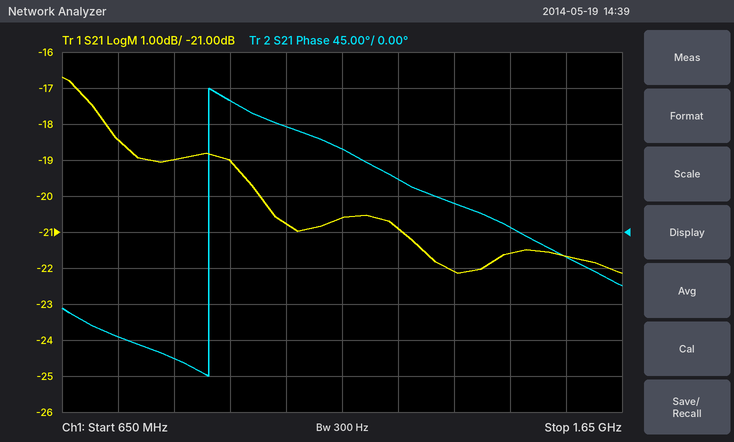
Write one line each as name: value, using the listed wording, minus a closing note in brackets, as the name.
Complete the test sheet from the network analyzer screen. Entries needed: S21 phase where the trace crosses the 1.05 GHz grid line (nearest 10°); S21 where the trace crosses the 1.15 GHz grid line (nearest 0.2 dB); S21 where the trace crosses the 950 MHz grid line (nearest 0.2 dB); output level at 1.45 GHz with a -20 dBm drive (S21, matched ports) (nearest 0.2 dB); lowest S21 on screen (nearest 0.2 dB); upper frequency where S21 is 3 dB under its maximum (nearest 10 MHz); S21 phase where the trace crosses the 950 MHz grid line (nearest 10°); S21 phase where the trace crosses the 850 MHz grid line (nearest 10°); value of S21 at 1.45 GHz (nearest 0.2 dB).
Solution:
S21 phase where the trace crosses the 1.05 GHz grid line: 130°
S21 where the trace crosses the 1.15 GHz grid line: -20.6 dB
S21 where the trace crosses the 950 MHz grid line: -19.0 dB
output level at 1.45 GHz with a -20 dBm drive (S21, matched ports): -41.6 dBm
lowest S21 on screen: -22.2 dB
upper frequency where S21 is 3 dB under its maximum: 990 MHz
S21 phase where the trace crosses the 950 MHz grid line: 160°
S21 phase where the trace crosses the 850 MHz grid line: -160°
value of S21 at 1.45 GHz: -21.6 dB
